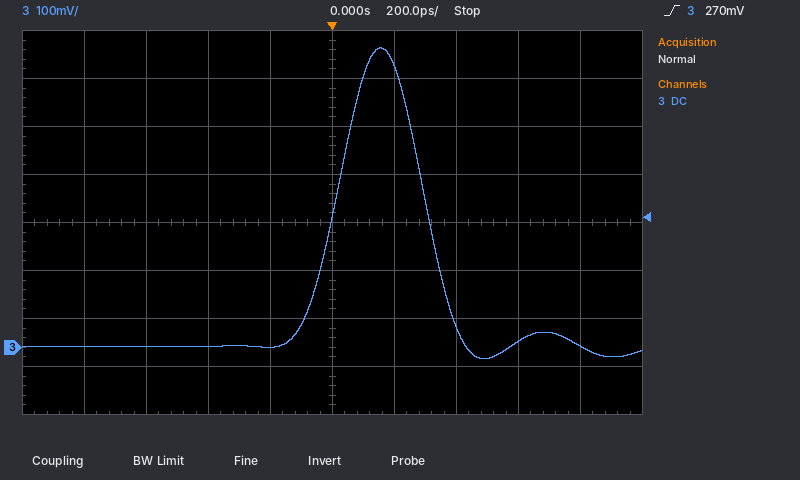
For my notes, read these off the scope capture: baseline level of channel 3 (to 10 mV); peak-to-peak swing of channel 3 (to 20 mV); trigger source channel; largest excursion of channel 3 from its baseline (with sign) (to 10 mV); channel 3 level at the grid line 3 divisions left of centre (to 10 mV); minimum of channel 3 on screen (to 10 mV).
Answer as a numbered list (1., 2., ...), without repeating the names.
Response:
1. 0 mV
2. 640 mV
3. channel 3
4. +620 mV
5. 0 mV
6. -20 mV
